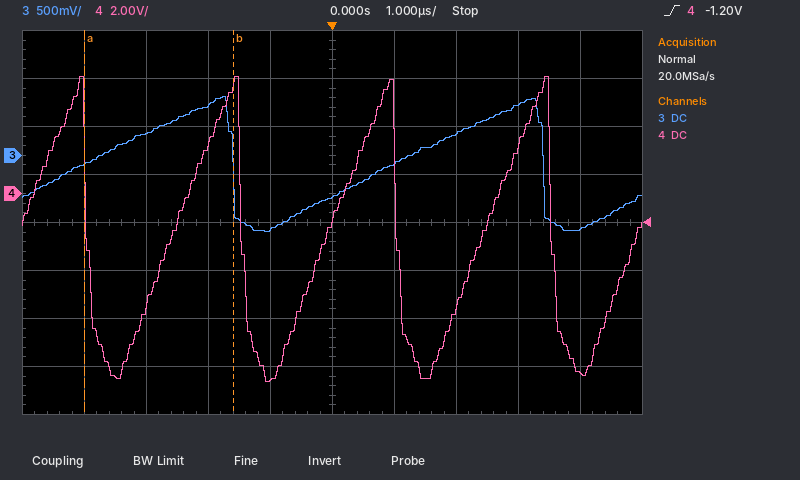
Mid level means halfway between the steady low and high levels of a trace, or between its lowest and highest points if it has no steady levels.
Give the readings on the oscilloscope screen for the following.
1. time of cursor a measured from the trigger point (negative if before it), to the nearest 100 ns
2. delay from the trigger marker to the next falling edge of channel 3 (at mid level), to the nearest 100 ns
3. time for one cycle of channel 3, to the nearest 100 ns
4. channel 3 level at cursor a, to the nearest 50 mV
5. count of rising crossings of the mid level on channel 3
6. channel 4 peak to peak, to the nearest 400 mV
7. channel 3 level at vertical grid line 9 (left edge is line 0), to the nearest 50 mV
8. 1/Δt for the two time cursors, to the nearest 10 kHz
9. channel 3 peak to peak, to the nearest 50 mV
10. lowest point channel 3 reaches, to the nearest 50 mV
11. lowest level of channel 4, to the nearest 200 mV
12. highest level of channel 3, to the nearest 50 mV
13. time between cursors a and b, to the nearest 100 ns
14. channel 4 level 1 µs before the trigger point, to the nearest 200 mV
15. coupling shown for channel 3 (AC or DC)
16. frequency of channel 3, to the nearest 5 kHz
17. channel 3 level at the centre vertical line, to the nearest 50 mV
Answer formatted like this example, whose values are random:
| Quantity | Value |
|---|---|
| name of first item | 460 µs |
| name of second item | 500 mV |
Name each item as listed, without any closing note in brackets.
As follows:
| Quantity | Value |
|---|---|
| time of cursor a measured from the trigger point (negative if before it), to the nearest 100 ns | -4.0 µs |
| delay from the trigger marker to the next falling edge of channel 3 (at mid level), to the nearest 100 ns | 3.4 µs |
| time for one cycle of channel 3, to the nearest 100 ns | 5.0 µs |
| channel 3 level at cursor a, to the nearest 50 mV | -100 mV |
| count of rising crossings of the mid level on channel 3 | 2 |
| channel 4 peak to peak, to the nearest 400 mV | 12.8 V |
| channel 3 level at vertical grid line 9 (left edge is line 0), to the nearest 50 mV | -750 mV |
| 1/Δt for the two time cursors, to the nearest 10 kHz | 420 kHz |
| channel 3 peak to peak, to the nearest 50 mV | 1.40 V |
| lowest point channel 3 reaches, to the nearest 50 mV | -800 mV |
| lowest level of channel 4, to the nearest 200 mV | -7.8 V |
| highest level of channel 3, to the nearest 50 mV | 600 mV |
| time between cursors a and b, to the nearest 100 ns | 2.4 µs |
| channel 4 level 1 µs before the trigger point, to the nearest 200 mV | -7.8 V |
| coupling shown for channel 3 | DC |
| frequency of channel 3, to the nearest 5 kHz | 200 kHz |
| channel 3 level at the centre vertical line, to the nearest 50 mV | -450 mV |
